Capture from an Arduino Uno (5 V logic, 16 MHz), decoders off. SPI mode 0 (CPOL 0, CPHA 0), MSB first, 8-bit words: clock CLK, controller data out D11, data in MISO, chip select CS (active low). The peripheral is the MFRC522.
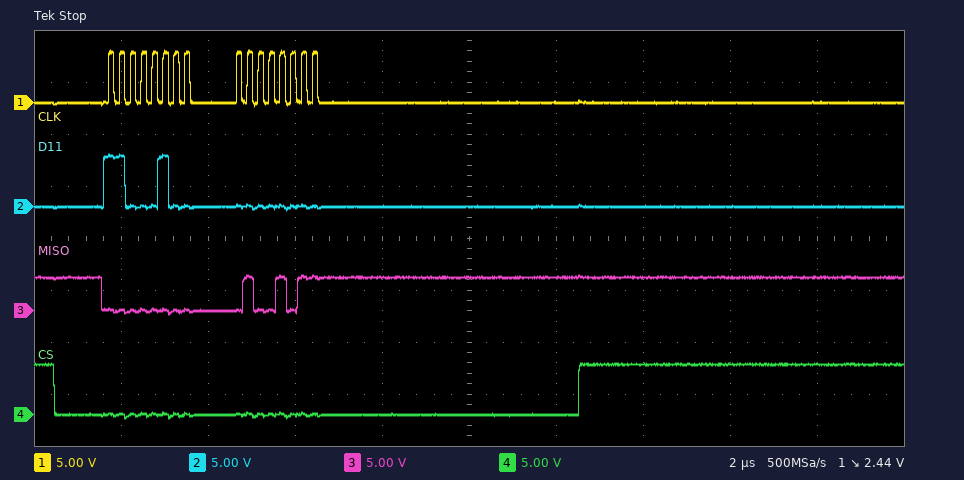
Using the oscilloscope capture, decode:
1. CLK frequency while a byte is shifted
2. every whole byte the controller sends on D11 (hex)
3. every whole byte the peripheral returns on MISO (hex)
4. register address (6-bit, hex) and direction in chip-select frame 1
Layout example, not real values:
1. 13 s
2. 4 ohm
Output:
1. 4 MHz
2. 0xC4 0x00
3. 0x00 0x4B
4. 0x22 read
